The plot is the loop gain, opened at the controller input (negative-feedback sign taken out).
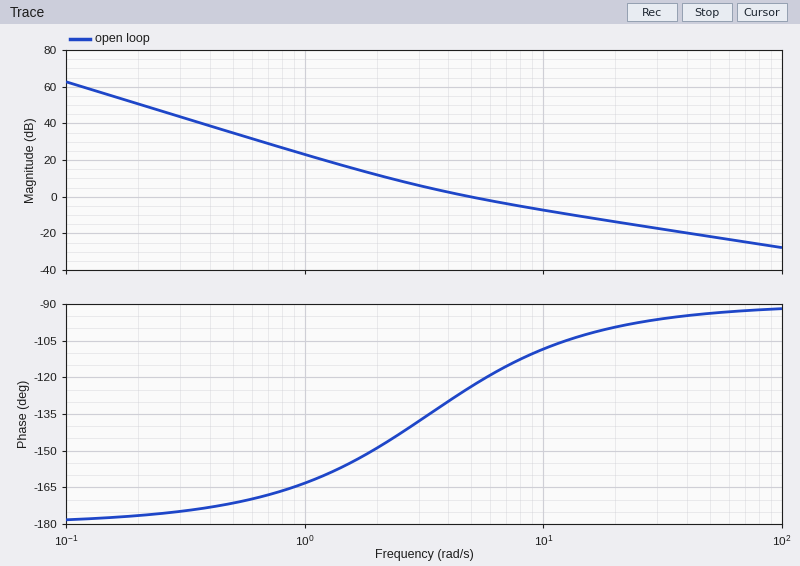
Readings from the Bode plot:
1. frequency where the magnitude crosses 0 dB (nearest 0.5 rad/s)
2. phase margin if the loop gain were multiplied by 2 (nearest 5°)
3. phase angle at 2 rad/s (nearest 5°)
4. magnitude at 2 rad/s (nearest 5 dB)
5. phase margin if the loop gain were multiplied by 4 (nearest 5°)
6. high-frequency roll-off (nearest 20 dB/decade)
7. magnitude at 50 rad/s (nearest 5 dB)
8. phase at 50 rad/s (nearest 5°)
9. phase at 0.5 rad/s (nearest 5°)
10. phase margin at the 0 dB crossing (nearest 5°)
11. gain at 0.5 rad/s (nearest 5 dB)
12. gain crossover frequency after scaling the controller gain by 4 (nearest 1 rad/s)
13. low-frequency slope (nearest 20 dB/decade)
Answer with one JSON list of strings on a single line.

["5.0 rad/s", "70°", "-150°", "10 dB", "80°", "-20 dB/decade", "-20 dB", "-95°", "-170°", "55°", "35 dB", "17 rad/s", "-40 dB/decade"]
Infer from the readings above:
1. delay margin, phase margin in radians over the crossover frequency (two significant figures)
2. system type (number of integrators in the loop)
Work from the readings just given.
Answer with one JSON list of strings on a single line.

["0.19 s", "2"]
